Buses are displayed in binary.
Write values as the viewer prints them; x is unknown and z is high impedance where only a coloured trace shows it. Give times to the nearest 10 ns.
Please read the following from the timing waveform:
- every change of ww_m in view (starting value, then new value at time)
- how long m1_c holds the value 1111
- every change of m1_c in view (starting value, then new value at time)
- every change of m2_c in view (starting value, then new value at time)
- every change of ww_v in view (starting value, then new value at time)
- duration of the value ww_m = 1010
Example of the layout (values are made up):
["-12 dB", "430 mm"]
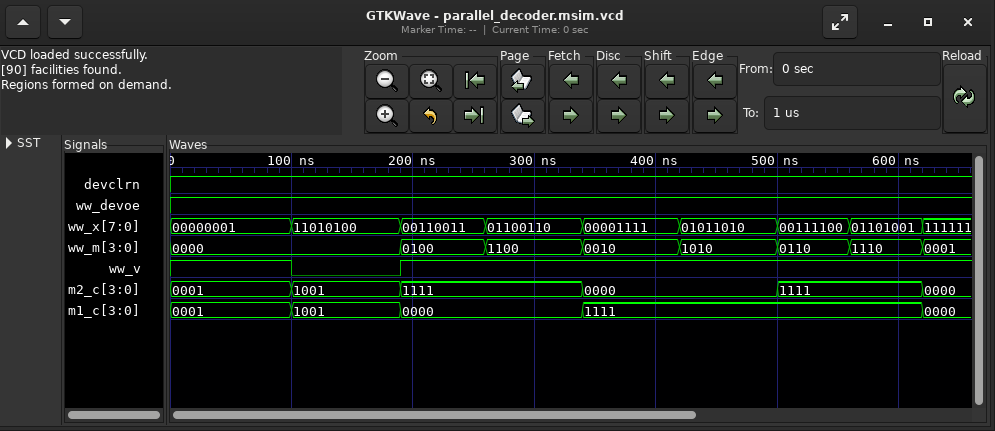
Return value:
["0000, 0100 at 190 ns, 1100 at 260 ns, 0010 at 340 ns, 1010 at 420 ns, 0110 at 500 ns, 1110 at 560 ns, 0001 at 620 ns", "280 ns", "0001, 1001 at 100 ns, 0000 at 190 ns, 1111 at 340 ns, 0000 at 620 ns", "0001, 1001 at 100 ns, 1111 at 190 ns, 0000 at 340 ns, 1111 at 500 ns, 0000 at 620 ns", "1, 0 at 100 ns, 1 at 190 ns", "80 ns"]
